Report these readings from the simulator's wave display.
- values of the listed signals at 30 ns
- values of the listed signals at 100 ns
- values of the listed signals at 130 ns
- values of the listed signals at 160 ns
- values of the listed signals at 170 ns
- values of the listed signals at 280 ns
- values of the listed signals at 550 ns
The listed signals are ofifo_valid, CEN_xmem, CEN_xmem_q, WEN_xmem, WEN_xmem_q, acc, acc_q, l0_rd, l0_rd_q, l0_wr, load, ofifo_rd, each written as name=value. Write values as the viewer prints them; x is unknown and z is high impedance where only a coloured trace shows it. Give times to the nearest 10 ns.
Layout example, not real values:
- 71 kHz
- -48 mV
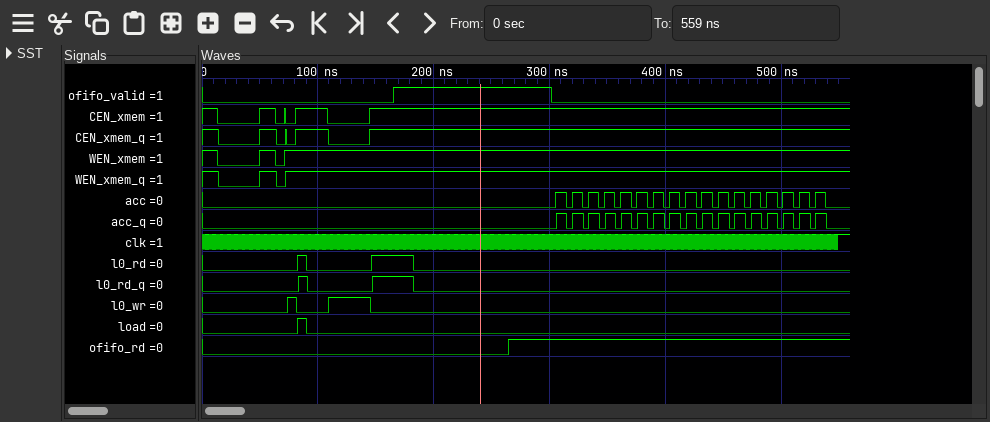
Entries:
- ofifo_valid=0, CEN_xmem=0, CEN_xmem_q=0, WEN_xmem=0, WEN_xmem_q=0, acc=0, acc_q=0, l0_rd=0, l0_rd_q=0, l0_wr=0, load=0, ofifo_rd=0
- ofifo_valid=0, CEN_xmem=1, CEN_xmem_q=1, WEN_xmem=1, WEN_xmem_q=1, acc=0, acc_q=0, l0_rd=0, l0_rd_q=0, l0_wr=0, load=0, ofifo_rd=0
- ofifo_valid=0, CEN_xmem=0, CEN_xmem_q=0, WEN_xmem=1, WEN_xmem_q=1, acc=0, acc_q=0, l0_rd=0, l0_rd_q=0, l0_wr=1, load=0, ofifo_rd=0
- ofifo_valid=0, CEN_xmem=1, CEN_xmem_q=1, WEN_xmem=1, WEN_xmem_q=1, acc=0, acc_q=0, l0_rd=1, l0_rd_q=1, l0_wr=0, load=0, ofifo_rd=0
- ofifo_valid=1, CEN_xmem=1, CEN_xmem_q=1, WEN_xmem=1, WEN_xmem_q=1, acc=0, acc_q=0, l0_rd=1, l0_rd_q=1, l0_wr=0, load=0, ofifo_rd=0
- ofifo_valid=1, CEN_xmem=1, CEN_xmem_q=1, WEN_xmem=1, WEN_xmem_q=1, acc=0, acc_q=0, l0_rd=0, l0_rd_q=0, l0_wr=0, load=0, ofifo_rd=1
- ofifo_valid=0, CEN_xmem=1, CEN_xmem_q=1, WEN_xmem=1, WEN_xmem_q=1, acc=0, acc_q=0, l0_rd=0, l0_rd_q=0, l0_wr=0, load=0, ofifo_rd=1
